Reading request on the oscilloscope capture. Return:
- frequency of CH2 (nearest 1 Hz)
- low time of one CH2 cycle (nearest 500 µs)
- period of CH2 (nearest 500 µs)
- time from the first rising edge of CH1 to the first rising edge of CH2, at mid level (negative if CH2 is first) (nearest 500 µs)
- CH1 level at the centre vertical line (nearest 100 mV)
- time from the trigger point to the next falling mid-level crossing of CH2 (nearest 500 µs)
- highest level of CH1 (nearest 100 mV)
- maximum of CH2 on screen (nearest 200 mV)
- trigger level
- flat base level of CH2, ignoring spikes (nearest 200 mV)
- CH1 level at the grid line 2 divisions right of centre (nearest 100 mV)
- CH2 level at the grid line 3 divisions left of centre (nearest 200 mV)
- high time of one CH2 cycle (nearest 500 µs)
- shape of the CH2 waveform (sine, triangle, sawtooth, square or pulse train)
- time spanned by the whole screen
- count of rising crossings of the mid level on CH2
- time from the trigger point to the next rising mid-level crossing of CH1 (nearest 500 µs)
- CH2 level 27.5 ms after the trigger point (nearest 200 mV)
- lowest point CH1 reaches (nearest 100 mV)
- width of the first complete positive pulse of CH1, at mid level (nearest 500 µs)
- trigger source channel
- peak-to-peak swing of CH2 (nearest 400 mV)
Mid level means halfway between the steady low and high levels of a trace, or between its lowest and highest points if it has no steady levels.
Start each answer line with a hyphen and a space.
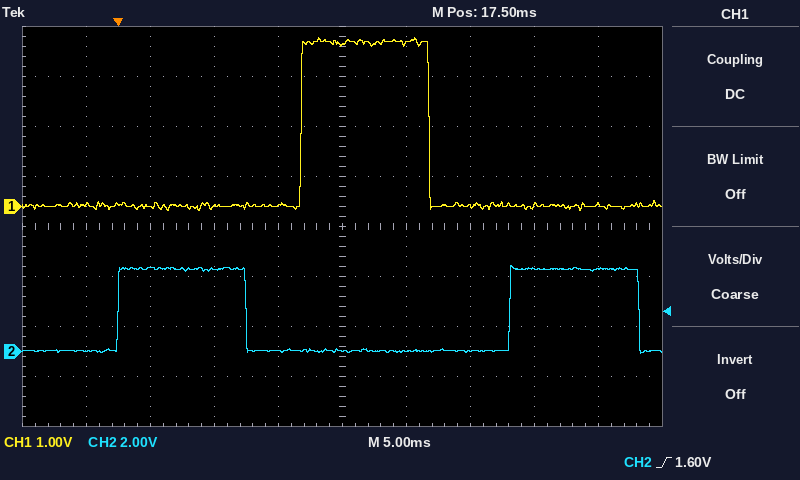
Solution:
- 33 Hz
- 20.5 ms
- 30.5 ms
- -14.5 ms
- 3.2 V
- 10.0 ms
- 3.4 V
- 3.4 V
- 1.60 V
- 0.0 V
- 0.0 V
- 3.4 V
- 10.0 ms
- pulse train
- 50 ms
- 2
- 14.5 ms
- 0.0 V
- -100 mV
- 10.0 ms
- CH2
- 3.6 V
